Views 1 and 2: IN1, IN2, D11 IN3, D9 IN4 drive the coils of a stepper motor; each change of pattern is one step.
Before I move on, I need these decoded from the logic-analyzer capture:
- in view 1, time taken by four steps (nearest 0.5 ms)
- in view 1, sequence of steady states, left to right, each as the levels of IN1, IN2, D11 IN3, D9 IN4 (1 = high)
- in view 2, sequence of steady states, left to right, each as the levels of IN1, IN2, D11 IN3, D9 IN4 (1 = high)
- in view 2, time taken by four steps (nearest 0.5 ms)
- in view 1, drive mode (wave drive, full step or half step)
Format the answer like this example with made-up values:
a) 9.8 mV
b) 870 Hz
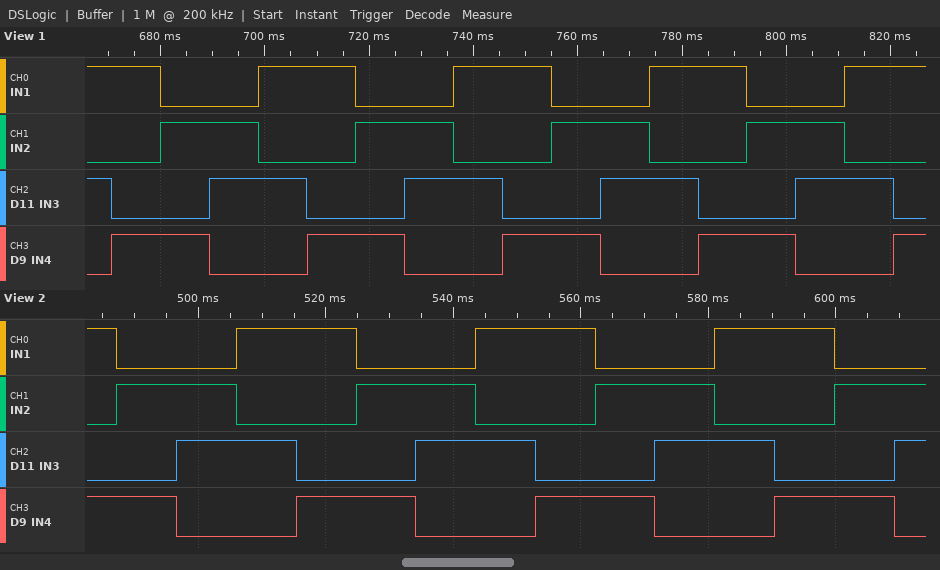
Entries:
a) 37.5 ms
b) 1010 1001 0101 0110 1010 1001 0101 0110 1010 1001 0101 0110 1010 1001 0101 0110 1010 1001
c) 1001 0101 0110 1010 1001 0101 0110 1010 1001 0101 0110 1010 1001 0101 0110
d) 37.5 ms
e) full step
